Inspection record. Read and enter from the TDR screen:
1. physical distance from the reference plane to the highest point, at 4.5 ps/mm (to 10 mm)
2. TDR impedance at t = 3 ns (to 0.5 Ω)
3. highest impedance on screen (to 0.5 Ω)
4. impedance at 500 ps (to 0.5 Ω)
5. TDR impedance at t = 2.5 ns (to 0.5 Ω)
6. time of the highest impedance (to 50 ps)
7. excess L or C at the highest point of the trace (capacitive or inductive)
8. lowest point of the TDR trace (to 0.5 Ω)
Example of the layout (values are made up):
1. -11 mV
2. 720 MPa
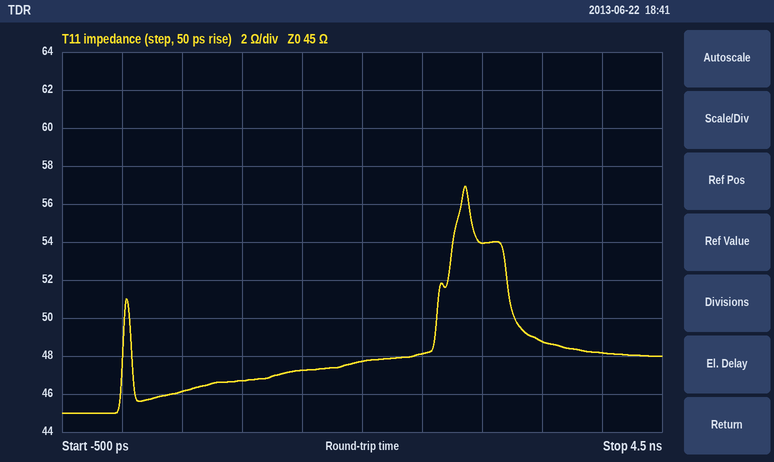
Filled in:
1. 320 mm
2. 54.0 Ω
3. 57.0 Ω
4. 46.0 Ω
5. 48.0 Ω
6. 2.85 ns
7. inductive
8. 45.0 Ω
